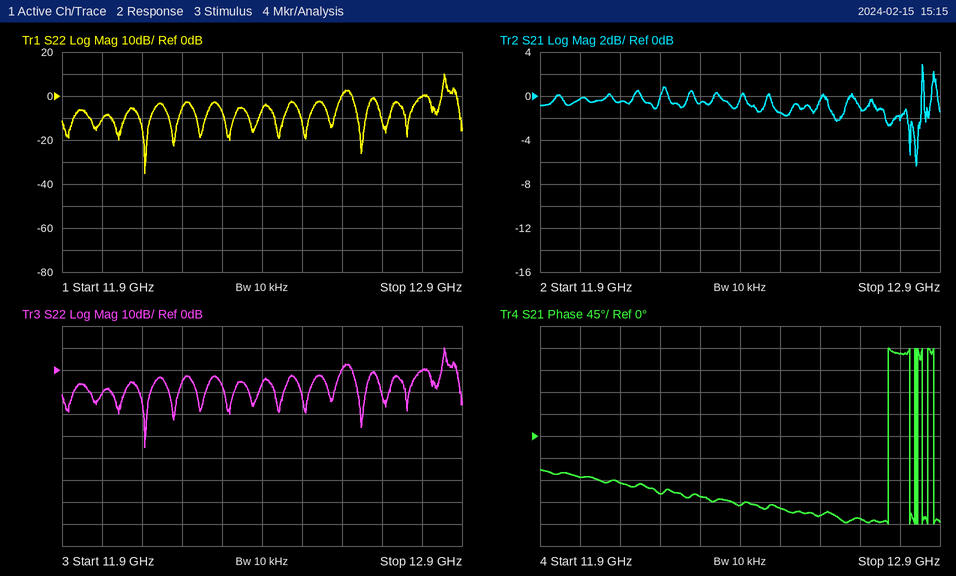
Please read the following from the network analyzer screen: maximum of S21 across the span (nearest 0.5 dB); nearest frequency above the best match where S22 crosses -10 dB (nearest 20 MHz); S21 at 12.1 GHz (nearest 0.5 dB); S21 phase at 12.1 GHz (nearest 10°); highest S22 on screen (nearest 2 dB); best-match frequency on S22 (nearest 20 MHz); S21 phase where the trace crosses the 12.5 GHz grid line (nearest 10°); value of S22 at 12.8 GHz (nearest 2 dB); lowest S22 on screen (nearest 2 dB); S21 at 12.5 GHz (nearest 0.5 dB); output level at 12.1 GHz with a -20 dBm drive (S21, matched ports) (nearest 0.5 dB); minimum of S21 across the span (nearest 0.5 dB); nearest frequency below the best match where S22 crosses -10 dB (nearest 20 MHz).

3.0 dB
12.12 GHz
-0.5 dB
-100°
10 dB
12.10 GHz
-150°
0 dB
-36 dB
-1.5 dB
-20.5 dBm
-6.5 dB
12.10 GHz
